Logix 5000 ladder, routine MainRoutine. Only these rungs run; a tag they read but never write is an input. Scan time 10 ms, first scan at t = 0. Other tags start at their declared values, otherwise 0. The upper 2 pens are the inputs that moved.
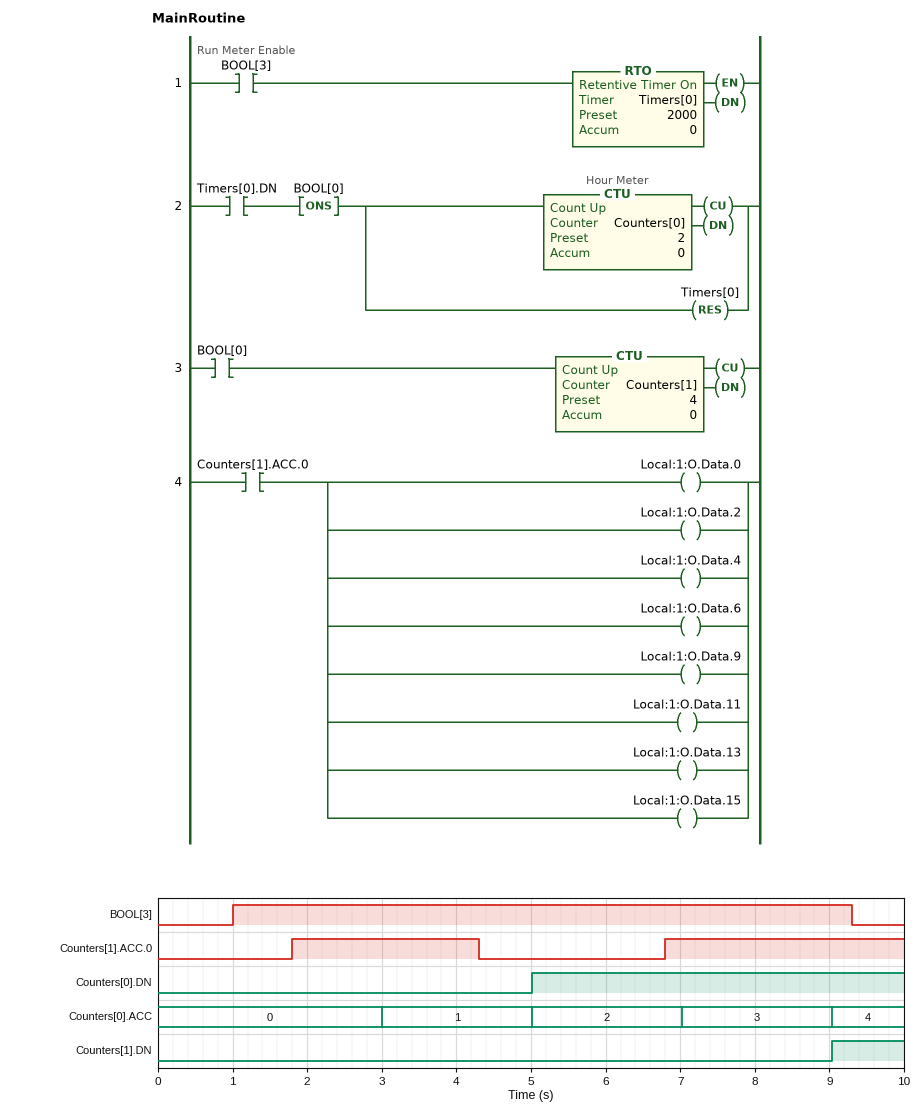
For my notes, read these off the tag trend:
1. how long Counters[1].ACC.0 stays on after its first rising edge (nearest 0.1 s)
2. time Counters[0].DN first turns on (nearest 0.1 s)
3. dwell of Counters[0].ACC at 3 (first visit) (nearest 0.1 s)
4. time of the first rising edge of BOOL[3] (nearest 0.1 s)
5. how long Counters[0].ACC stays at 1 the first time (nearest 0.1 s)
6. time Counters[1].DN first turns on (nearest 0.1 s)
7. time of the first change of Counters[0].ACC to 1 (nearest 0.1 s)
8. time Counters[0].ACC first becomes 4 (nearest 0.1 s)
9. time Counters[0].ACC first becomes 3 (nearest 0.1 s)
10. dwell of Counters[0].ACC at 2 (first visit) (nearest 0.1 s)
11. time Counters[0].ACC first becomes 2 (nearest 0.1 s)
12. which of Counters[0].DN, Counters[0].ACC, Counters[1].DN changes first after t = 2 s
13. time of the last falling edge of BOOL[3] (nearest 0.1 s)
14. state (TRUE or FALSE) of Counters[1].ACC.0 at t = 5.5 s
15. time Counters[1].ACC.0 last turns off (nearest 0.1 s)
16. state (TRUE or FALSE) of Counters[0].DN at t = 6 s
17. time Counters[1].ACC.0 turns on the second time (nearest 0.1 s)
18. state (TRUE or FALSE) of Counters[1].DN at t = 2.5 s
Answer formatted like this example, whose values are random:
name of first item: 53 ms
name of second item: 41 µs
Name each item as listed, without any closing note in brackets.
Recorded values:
how long Counters[1].ACC.0 stays on after its first rising edge: 2.5 s
time Counters[0].DN first turns on: 5.0 s
dwell of Counters[0].ACC at 3 (first visit): 2.0 s
time of the first rising edge of BOOL[3]: 1.0 s
how long Counters[0].ACC stays at 1 the first time: 2.0 s
time Counters[1].DN first turns on: 9.0 s
time of the first change of Counters[0].ACC to 1: 3.0 s
time Counters[0].ACC first becomes 4: 9.0 s
time Counters[0].ACC first becomes 3: 7.0 s
dwell of Counters[0].ACC at 2 (first visit): 2.0 s
time Counters[0].ACC first becomes 2: 5.0 s
which of Counters[0].DN, Counters[0].ACC, Counters[1].DN changes first after t = 2 s: Counters[0].ACC
time of the last falling edge of BOOL[3]: 9.3 s
state (TRUE or FALSE) of Counters[1].ACC.0 at t = 5.5 s: FALSE
time Counters[1].ACC.0 last turns off: 4.3 s
state (TRUE or FALSE) of Counters[0].DN at t = 6 s: TRUE
time Counters[1].ACC.0 turns on the second time: 6.8 s
state (TRUE or FALSE) of Counters[1].DN at t = 2.5 s: FALSE
